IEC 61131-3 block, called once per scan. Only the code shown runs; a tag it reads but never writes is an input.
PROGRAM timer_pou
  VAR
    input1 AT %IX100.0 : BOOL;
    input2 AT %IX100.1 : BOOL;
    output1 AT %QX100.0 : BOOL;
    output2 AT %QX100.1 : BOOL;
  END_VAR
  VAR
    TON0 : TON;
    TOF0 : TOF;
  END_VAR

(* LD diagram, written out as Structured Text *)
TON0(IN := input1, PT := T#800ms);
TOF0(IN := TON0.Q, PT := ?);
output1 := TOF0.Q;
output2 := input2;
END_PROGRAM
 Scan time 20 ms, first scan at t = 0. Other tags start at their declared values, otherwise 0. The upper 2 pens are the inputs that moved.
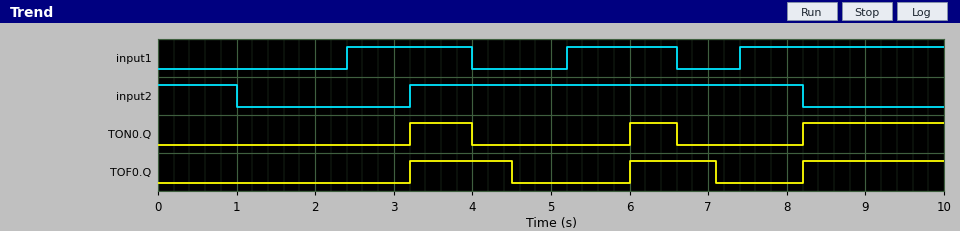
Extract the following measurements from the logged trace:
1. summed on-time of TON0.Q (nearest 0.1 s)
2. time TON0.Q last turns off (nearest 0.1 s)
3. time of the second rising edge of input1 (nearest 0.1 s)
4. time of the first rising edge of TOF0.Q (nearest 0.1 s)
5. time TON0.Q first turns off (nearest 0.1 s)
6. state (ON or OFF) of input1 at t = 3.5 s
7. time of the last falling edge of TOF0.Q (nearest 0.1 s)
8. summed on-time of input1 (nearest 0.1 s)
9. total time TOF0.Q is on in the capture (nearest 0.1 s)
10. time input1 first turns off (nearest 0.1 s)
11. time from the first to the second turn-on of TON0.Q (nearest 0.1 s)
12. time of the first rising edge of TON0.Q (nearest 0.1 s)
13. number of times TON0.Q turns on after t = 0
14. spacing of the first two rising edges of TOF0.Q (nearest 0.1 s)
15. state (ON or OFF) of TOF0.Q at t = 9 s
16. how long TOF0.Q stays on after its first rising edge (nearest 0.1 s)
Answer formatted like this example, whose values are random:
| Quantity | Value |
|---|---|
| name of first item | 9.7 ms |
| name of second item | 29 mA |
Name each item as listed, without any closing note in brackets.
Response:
| Quantity | Value |
|---|---|
| summed on-time of TON0.Q | 3.2 s |
| time TON0.Q last turns off | 6.6 s |
| time of the second rising edge of input1 | 5.2 s |
| time of the first rising edge of TOF0.Q | 3.2 s |
| time TON0.Q first turns off | 4.0 s |
| state (ON or OFF) of input1 at t = 3.5 s | ON |
| time of the last falling edge of TOF0.Q | 7.1 s |
| summed on-time of input1 | 5.6 s |
| total time TOF0.Q is on in the capture | 4.2 s |
| time input1 first turns off | 4.0 s |
| time from the first to the second turn-on of TON0.Q | 2.8 s |
| time of the first rising edge of TON0.Q | 3.2 s |
| number of times TON0.Q turns on after t = 0 | 3 |
| spacing of the first two rising edges of TOF0.Q | 2.8 s |
| state (ON or OFF) of TOF0.Q at t = 9 s | ON |
| how long TOF0.Q stays on after its first rising edge | 1.3 s |
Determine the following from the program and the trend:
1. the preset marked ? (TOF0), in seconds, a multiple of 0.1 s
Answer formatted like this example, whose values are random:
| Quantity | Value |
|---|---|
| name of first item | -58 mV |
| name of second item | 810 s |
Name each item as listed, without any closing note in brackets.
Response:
| Quantity | Value |
|---|---|
| the preset marked ? (TOF0), in seconds, a multiple of 0.1 s | 0.5 s |
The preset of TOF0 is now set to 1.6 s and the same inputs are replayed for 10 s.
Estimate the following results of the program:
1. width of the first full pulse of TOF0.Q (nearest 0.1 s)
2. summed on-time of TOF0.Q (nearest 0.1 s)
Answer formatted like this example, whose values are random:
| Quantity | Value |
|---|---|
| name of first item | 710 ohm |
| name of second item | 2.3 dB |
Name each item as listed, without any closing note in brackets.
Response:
| Quantity | Value |
|---|---|
| width of the first full pulse of TOF0.Q | 2.4 s |
| summed on-time of TOF0.Q | 6.4 s |
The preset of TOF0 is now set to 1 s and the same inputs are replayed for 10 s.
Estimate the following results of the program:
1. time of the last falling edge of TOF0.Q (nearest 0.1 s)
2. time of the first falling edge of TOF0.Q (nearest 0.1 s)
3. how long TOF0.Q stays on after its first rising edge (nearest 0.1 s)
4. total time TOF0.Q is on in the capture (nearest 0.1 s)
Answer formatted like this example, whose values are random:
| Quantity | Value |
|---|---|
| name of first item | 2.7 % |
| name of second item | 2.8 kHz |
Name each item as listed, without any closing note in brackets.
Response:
| Quantity | Value |
|---|---|
| time of the last falling edge of TOF0.Q | 7.6 s |
| time of the first falling edge of TOF0.Q | 5.0 s |
| how long TOF0.Q stays on after its first rising edge | 1.8 s |
| total time TOF0.Q is on in the capture | 5.2 s |
